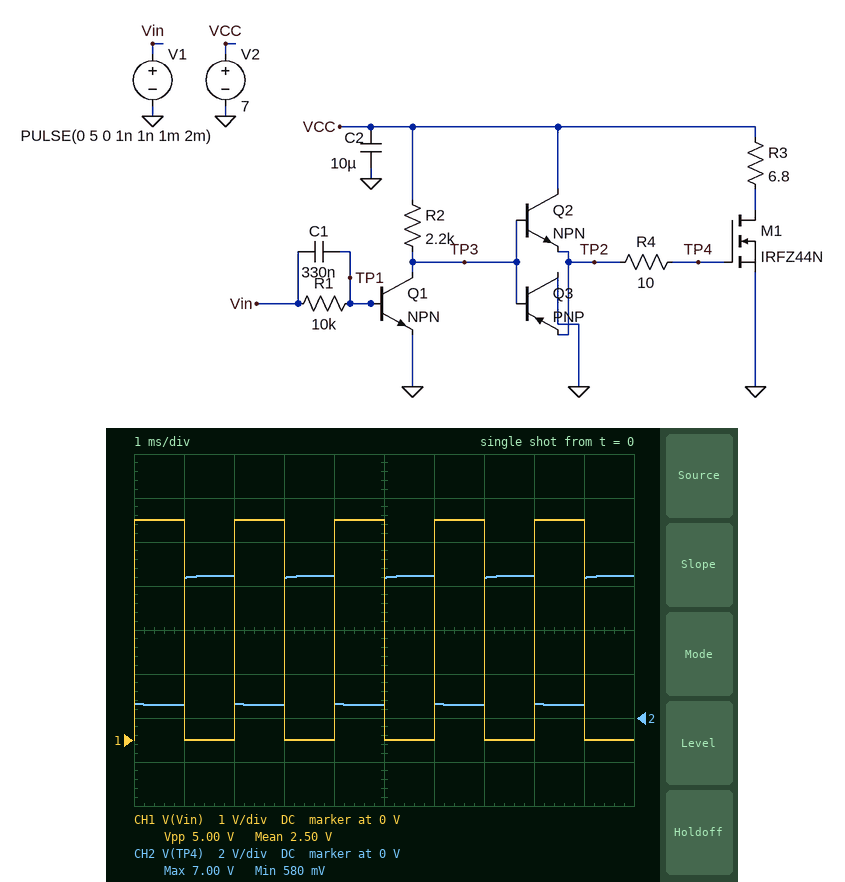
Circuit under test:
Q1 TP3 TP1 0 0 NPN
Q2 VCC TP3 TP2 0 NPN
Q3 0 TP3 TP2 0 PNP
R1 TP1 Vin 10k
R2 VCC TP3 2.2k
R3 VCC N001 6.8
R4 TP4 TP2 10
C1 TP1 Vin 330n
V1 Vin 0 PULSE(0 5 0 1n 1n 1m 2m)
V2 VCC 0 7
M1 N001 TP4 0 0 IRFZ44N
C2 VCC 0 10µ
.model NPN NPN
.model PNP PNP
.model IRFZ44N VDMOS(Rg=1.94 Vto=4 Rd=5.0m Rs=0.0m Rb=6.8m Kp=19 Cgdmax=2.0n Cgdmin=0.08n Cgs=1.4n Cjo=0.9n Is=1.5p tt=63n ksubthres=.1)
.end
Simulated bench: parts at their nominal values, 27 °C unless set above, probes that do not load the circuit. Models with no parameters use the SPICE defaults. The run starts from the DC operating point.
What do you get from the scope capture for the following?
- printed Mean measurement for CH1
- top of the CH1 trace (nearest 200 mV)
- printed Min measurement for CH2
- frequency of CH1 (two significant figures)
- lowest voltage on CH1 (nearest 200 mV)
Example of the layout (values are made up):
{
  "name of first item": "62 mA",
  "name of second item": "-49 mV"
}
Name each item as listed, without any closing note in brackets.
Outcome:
{
  "printed Mean measurement for CH1": "2.50 V",
  "top of the CH1 trace": "5.0 V",
  "printed Min measurement for CH2": "580 mV",
  "frequency of CH1": "500 Hz",
  "lowest voltage on CH1": "0 V"
}
